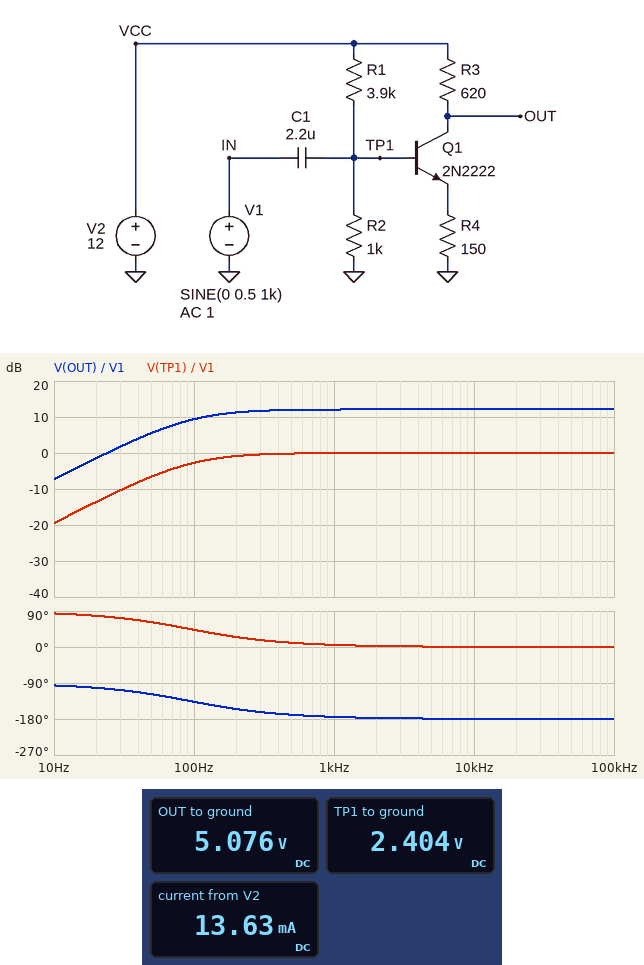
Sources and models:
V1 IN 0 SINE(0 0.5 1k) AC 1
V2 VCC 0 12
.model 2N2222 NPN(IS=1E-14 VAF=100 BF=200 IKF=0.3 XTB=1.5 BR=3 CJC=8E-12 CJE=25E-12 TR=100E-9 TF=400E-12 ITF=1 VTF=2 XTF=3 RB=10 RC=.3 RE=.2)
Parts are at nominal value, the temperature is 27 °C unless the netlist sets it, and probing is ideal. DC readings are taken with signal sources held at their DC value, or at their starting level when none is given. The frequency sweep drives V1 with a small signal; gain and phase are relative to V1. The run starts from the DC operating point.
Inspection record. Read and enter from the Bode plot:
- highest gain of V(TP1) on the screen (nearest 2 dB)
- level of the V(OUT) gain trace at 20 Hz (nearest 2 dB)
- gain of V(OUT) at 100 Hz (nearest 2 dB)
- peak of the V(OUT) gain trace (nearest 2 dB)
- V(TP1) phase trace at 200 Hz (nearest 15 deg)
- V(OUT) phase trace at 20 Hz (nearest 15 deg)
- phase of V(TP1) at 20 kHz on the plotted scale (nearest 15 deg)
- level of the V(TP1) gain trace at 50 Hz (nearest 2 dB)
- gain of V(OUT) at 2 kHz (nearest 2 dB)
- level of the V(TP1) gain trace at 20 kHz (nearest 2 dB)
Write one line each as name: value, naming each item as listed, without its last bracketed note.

highest gain of V(TP1) on the screen: 0 dB
level of the V(OUT) gain trace at 20 Hz: -2 dB
gain of V(OUT) at 100 Hz: 10 dB
peak of the V(OUT) gain trace: 12 dB
V(TP1) phase trace at 200 Hz: 30 deg
V(OUT) phase trace at 20 Hz: -105 deg
phase of V(TP1) at 20 kHz on the plotted scale: 0 deg
level of the V(TP1) gain trace at 50 Hz: -6 dB
gain of V(OUT) at 2 kHz: 12 dB
level of the V(TP1) gain trace at 20 kHz: 0 dB
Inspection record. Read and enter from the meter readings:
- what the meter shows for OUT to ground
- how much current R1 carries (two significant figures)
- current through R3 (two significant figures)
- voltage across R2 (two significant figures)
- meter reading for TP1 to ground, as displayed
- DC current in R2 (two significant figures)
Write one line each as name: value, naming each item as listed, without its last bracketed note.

what the meter shows for OUT to ground: 5.076 V
how much current R1 carries: 2.5 mA
current through R3: 11 mA
voltage across R2: 2.4 V
meter reading for TP1 to ground, as displayed: 2.404 V
DC current in R2: 2.4 mA
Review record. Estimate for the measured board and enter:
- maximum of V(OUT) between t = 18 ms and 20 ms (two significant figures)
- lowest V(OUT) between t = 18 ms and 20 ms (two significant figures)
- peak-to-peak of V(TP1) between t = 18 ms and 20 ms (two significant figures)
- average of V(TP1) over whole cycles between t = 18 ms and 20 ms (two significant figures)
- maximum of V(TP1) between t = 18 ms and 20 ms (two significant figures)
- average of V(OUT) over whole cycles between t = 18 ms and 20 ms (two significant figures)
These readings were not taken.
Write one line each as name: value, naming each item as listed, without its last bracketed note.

maximum of V(OUT) between t = 18 ms and 20 ms: 7.1 V
lowest V(OUT) between t = 18 ms and 20 ms: 3.1 V
peak-to-peak of V(TP1) between t = 18 ms and 20 ms: 1.0 V
average of V(TP1) over whole cycles between t = 18 ms and 20 ms: 2.4 V
maximum of V(TP1) between t = 18 ms and 20 ms: 2.9 V
average of V(OUT) over whole cycles between t = 18 ms and 20 ms: 5.1 V
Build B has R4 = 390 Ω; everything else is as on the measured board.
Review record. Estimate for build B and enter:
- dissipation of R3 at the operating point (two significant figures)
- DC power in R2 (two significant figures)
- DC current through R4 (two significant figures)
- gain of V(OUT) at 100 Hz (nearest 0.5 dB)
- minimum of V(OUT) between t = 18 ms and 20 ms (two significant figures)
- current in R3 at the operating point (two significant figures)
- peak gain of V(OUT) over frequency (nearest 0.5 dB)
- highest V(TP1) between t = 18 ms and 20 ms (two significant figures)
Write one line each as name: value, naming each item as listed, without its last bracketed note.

dissipation of R3 at the operating point: 12 mW
DC power in R2: 5.9 mW
DC current through R4: 4.5 mA
gain of V(OUT) at 100 Hz: 1.0 dB
minimum of V(OUT) between t = 18 ms and 20 ms: 8.5 V
current in R3 at the operating point: 4.4 mA
peak gain of V(OUT) over frequency: 4.0 dB
highest V(TP1) between t = 18 ms and 20 ms: 2.9 V
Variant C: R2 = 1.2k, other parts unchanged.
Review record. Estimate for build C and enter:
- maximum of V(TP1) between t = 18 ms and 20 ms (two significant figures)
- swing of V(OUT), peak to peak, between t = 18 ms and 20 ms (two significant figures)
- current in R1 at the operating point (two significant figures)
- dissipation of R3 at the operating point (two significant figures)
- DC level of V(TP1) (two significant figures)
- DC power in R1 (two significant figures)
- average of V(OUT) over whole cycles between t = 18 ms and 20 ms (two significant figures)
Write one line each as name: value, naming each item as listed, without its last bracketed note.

maximum of V(TP1) between t = 18 ms and 20 ms: 3.2 V
swing of V(OUT), peak to peak, between t = 18 ms and 20 ms: 3.6 V
current in R1 at the operating point: 2.4 mA
dissipation of R3 at the operating point: 110 mW
DC level of V(TP1): 2.8 V
DC power in R1: 22 mW
average of V(OUT) over whole cycles between t = 18 ms and 20 ms: 4.1 V
